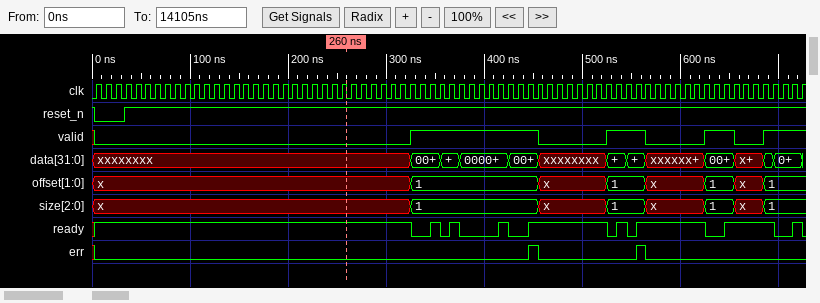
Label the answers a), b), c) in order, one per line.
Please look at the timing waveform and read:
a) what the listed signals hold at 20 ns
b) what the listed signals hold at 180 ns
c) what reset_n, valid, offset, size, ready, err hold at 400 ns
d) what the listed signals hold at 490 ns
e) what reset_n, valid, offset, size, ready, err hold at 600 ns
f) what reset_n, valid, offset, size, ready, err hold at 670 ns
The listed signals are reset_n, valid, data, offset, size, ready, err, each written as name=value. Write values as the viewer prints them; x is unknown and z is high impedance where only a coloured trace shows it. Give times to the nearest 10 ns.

a) reset_n=0, valid=0, data=xxxxxxxx, offset=x, size=x, ready=1, err=0
b) reset_n=1, valid=0, data=xxxxxxxx, offset=x, size=x, ready=1, err=0
c) reset_n=1, valid=1, offset=1, size=1, ready=0, err=0
d) reset_n=1, valid=0, data=xxxxxxxx, offset=x, size=x, ready=1, err=0
e) reset_n=1, valid=0, offset=x, size=x, ready=1, err=0
f) reset_n=1, valid=0, offset=x, size=x, ready=1, err=0
